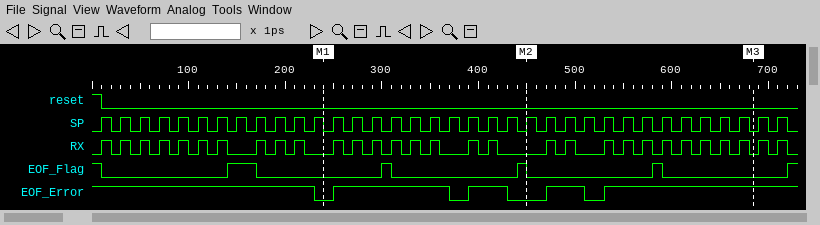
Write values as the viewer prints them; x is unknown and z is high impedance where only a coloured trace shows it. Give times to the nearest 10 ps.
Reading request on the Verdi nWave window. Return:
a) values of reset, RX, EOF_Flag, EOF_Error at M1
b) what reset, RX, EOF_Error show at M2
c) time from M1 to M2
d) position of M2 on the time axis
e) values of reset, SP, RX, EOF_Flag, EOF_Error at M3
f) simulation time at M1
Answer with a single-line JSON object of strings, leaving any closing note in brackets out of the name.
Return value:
{"values of reset, RX, EOF_Flag, EOF_Error at M1": "reset=0, RX=0, EOF_Flag=0, EOF_Error=0", "what reset, RX, EOF_Error show at M2": "reset=0, RX=0, EOF_Error=0", "time from M1 to M2": "210 ps", "position of M2 on the time axis": "450 ps", "values of reset, SP, RX, EOF_Flag, EOF_Error at M3": "reset=0, SP=0, RX=0, EOF_Flag=0, EOF_Error=1", "simulation time at M1": "240 ps"}
